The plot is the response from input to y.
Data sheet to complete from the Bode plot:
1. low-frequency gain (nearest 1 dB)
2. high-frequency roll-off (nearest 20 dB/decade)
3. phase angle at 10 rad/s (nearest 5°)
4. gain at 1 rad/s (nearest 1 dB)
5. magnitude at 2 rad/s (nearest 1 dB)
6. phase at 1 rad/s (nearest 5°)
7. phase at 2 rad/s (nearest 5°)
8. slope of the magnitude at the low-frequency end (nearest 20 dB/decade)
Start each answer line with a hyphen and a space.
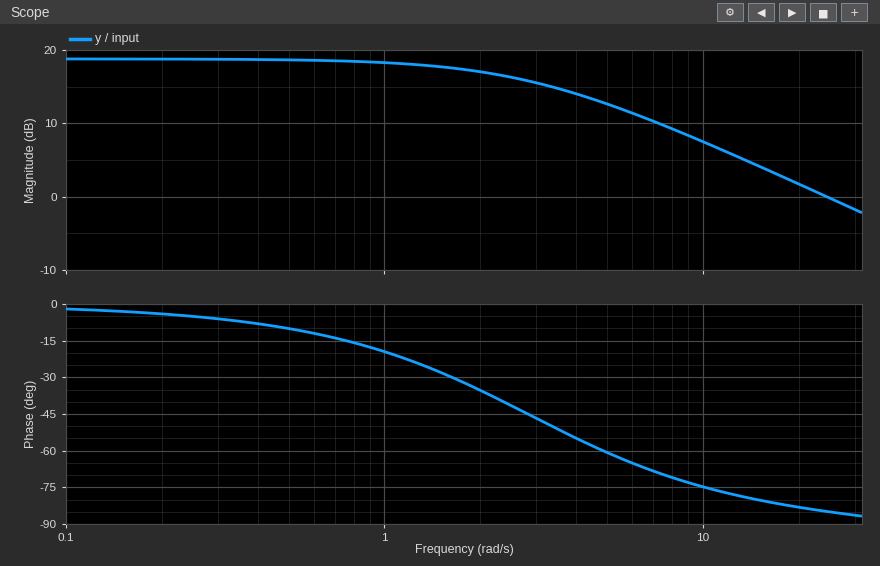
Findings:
- 19 dB
- -20 dB/decade
- -75°
- 18 dB
- 17 dB
- -20°
- -35°
- 0 dB/decade
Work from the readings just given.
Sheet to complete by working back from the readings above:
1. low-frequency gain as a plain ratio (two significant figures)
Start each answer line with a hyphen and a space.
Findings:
- 8.9
